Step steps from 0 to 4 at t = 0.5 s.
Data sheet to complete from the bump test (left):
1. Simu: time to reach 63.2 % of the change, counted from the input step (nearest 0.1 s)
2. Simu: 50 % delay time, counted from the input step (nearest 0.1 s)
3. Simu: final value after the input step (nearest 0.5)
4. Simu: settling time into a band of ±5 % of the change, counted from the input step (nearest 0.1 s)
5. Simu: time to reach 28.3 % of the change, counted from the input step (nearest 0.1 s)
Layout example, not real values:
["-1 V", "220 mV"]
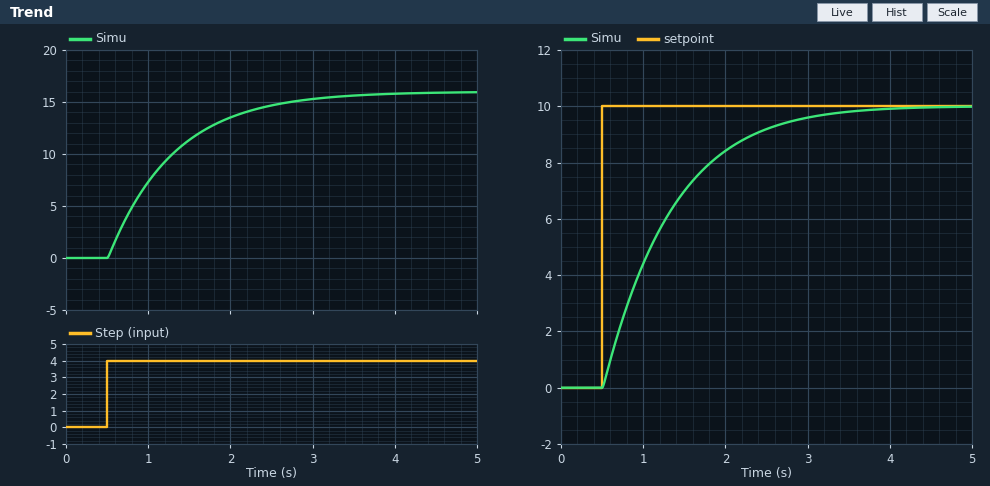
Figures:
["0.8 s", "0.6 s", "16.0", "2.4 s", "0.3 s"]
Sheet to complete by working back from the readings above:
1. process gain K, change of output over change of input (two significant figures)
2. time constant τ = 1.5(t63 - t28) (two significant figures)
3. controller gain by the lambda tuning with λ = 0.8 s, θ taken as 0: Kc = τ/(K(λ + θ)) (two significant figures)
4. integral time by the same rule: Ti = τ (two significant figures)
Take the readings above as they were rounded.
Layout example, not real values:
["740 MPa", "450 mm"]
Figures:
["4.0", "0.75 s", "0.23", "0.75 s"]
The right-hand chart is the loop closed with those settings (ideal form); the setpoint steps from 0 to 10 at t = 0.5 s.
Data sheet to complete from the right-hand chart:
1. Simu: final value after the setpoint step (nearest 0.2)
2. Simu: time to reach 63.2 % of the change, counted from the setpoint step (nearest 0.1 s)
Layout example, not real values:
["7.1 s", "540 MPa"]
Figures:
["10.0", "0.8 s"]
